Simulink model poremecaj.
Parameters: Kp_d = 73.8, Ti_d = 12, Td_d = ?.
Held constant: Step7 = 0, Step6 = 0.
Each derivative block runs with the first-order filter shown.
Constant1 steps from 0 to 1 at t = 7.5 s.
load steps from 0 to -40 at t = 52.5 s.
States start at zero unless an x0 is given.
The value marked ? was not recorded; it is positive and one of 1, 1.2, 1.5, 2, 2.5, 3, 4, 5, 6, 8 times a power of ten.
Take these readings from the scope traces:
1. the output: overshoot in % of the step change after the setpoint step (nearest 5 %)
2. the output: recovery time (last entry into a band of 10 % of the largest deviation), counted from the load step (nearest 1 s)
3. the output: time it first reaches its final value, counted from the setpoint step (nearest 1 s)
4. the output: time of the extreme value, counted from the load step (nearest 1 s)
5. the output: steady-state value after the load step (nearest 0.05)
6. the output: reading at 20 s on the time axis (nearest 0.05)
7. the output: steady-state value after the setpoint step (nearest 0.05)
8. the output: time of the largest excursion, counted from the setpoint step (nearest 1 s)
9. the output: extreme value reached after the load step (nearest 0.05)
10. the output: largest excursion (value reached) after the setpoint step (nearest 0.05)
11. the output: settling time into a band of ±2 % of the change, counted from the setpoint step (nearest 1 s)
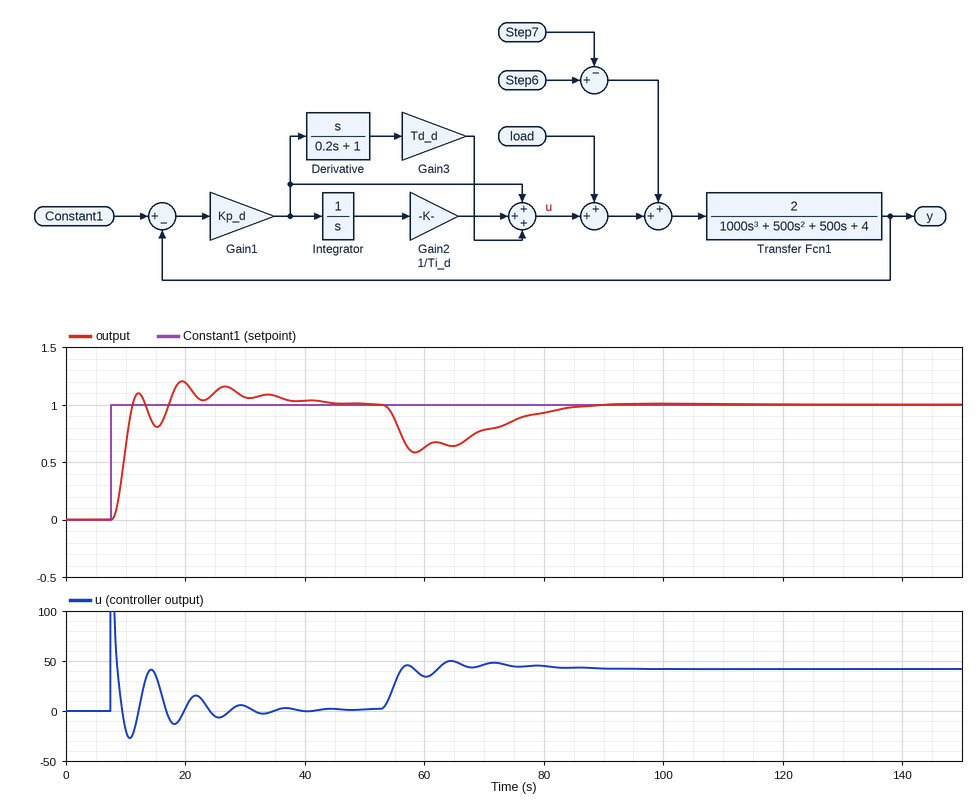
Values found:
20 %
30 s
4 s
6 s
1.00
1.20
1.00
12 s
0.60
1.20
36 s
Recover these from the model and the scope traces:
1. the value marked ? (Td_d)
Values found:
2
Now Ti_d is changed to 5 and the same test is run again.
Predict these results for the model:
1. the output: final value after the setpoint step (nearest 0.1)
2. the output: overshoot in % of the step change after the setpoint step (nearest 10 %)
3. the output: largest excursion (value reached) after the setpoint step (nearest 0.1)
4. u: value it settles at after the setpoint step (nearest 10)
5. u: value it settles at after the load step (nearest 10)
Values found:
1.0
30 %
1.3
0
40
